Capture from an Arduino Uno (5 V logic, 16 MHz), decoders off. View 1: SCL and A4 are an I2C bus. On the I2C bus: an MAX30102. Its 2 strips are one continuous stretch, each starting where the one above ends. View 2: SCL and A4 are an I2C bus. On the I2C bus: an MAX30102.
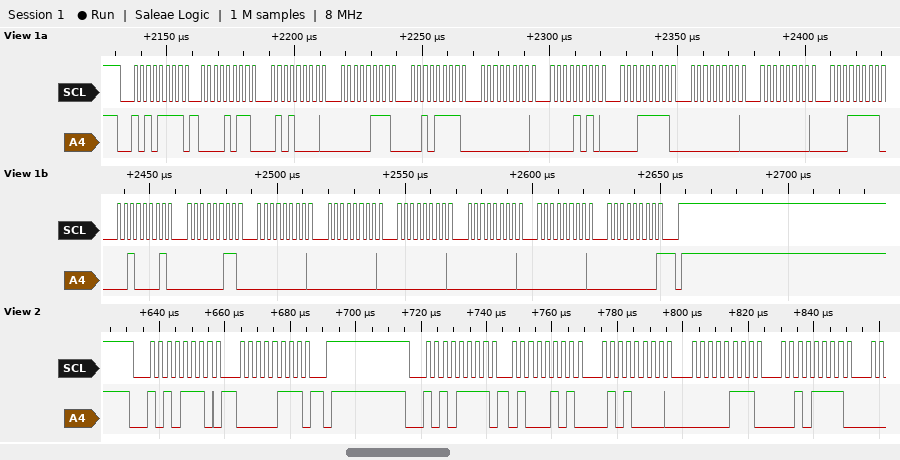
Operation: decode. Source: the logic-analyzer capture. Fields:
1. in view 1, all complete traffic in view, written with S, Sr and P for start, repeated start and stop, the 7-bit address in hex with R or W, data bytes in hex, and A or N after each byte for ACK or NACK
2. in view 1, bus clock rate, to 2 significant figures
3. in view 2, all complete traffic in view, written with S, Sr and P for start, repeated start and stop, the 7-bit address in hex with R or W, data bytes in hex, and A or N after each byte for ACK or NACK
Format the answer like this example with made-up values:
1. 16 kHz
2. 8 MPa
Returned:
1. S 57R A 0B A 50 A 07 A 2F A 00 A 0A A 1F A 00 A 00 A 1F A 21 A 03 A 00 A 00 A 00 A 00 A 00 A 00 N P
2. 400 kHz
3. S 57W A 07 A P S 57R A 45 A 50 A 07 A 2F A
